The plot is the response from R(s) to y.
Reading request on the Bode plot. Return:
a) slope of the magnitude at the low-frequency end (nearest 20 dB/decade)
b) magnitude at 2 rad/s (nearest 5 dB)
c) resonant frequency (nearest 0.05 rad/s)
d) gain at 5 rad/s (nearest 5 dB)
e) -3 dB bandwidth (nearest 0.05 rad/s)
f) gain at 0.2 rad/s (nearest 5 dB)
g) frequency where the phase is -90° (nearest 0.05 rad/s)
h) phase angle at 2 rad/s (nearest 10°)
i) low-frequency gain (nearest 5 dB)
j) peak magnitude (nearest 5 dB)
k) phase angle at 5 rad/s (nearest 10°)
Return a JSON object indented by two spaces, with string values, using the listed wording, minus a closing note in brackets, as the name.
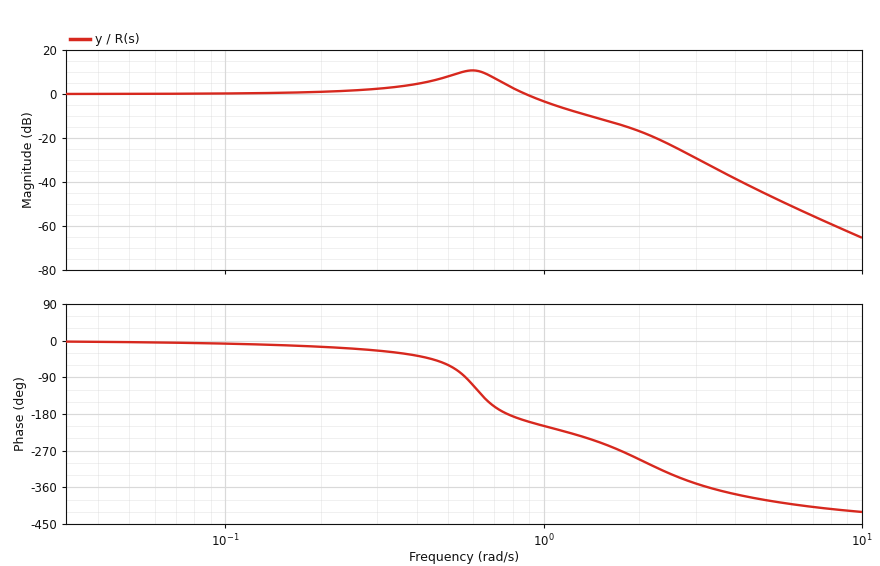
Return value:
{
  "slope of the magnitude at the low-frequency end": "0 dB/decade",
  "magnitude at 2 rad/s": "-15 dB",
  "resonant frequency": "0.60 rad/s",
  "gain at 5 rad/s": "-45 dB",
  "-3 dB bandwidth": "1.00 rad/s",
  "gain at 0.2 rad/s": "0 dB",
  "frequency where the phase is -90°": "0.55 rad/s",
  "phase angle at 2 rad/s": "-290°",
  "low-frequency gain": "0 dB",
  "peak magnitude": "10 dB",
  "phase angle at 5 rad/s": "-390°"
}
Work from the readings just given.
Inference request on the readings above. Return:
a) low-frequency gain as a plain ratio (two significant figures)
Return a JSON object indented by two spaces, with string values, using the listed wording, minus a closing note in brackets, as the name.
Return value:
{
  "low-frequency gain as a plain ratio": "1.0"
}
